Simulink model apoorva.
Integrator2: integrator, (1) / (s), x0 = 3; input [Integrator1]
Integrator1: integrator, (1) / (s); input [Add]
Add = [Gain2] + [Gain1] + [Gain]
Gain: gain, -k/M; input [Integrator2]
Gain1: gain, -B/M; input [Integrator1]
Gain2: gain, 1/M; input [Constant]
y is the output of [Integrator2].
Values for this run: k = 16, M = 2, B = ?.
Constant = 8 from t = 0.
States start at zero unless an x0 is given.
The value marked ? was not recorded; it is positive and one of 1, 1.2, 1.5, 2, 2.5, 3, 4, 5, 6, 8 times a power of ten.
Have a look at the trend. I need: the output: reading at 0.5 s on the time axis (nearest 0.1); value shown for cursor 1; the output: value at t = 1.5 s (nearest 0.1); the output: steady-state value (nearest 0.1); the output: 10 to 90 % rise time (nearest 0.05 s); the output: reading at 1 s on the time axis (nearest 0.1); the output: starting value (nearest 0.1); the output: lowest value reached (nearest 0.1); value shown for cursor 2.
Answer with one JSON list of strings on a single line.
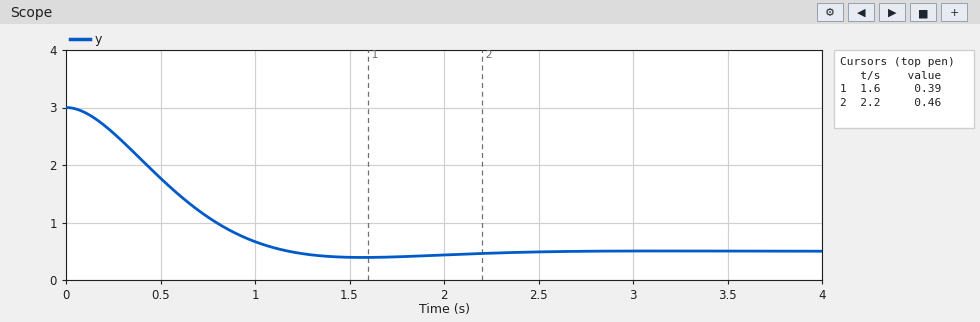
["1.8", "0.39", "0.4", "0.5", "0.75 s", "0.7", "3.0", "0.4", "0.46"]
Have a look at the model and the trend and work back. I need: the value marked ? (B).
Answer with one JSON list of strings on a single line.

["8"]
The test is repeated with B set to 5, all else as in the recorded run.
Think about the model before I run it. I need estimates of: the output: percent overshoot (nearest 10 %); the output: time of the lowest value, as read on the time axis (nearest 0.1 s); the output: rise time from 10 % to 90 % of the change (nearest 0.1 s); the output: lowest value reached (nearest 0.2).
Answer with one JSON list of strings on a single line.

["20 %", "1.2 s", "0.5 s", "0.0"]
